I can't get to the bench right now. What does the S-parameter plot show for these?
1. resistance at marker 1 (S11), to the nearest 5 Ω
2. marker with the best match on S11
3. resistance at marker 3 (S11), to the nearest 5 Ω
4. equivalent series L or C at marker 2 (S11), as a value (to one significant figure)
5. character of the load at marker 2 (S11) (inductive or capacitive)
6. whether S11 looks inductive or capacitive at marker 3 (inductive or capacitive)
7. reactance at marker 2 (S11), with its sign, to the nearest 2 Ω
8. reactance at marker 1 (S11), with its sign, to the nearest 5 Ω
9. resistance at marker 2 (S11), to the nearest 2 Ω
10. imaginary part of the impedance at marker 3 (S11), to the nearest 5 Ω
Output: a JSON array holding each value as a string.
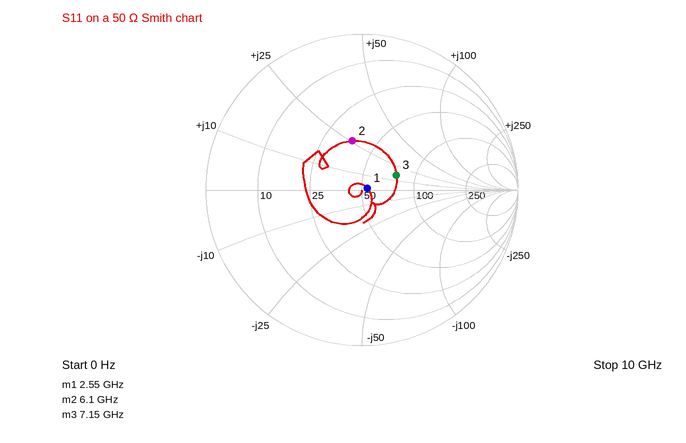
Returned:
["55 Ω", "marker 1", "75 Ω", "700 pH", "inductive", "inductive", "+26 Ω", "0 Ω", "36 Ω", "+15 Ω"]
